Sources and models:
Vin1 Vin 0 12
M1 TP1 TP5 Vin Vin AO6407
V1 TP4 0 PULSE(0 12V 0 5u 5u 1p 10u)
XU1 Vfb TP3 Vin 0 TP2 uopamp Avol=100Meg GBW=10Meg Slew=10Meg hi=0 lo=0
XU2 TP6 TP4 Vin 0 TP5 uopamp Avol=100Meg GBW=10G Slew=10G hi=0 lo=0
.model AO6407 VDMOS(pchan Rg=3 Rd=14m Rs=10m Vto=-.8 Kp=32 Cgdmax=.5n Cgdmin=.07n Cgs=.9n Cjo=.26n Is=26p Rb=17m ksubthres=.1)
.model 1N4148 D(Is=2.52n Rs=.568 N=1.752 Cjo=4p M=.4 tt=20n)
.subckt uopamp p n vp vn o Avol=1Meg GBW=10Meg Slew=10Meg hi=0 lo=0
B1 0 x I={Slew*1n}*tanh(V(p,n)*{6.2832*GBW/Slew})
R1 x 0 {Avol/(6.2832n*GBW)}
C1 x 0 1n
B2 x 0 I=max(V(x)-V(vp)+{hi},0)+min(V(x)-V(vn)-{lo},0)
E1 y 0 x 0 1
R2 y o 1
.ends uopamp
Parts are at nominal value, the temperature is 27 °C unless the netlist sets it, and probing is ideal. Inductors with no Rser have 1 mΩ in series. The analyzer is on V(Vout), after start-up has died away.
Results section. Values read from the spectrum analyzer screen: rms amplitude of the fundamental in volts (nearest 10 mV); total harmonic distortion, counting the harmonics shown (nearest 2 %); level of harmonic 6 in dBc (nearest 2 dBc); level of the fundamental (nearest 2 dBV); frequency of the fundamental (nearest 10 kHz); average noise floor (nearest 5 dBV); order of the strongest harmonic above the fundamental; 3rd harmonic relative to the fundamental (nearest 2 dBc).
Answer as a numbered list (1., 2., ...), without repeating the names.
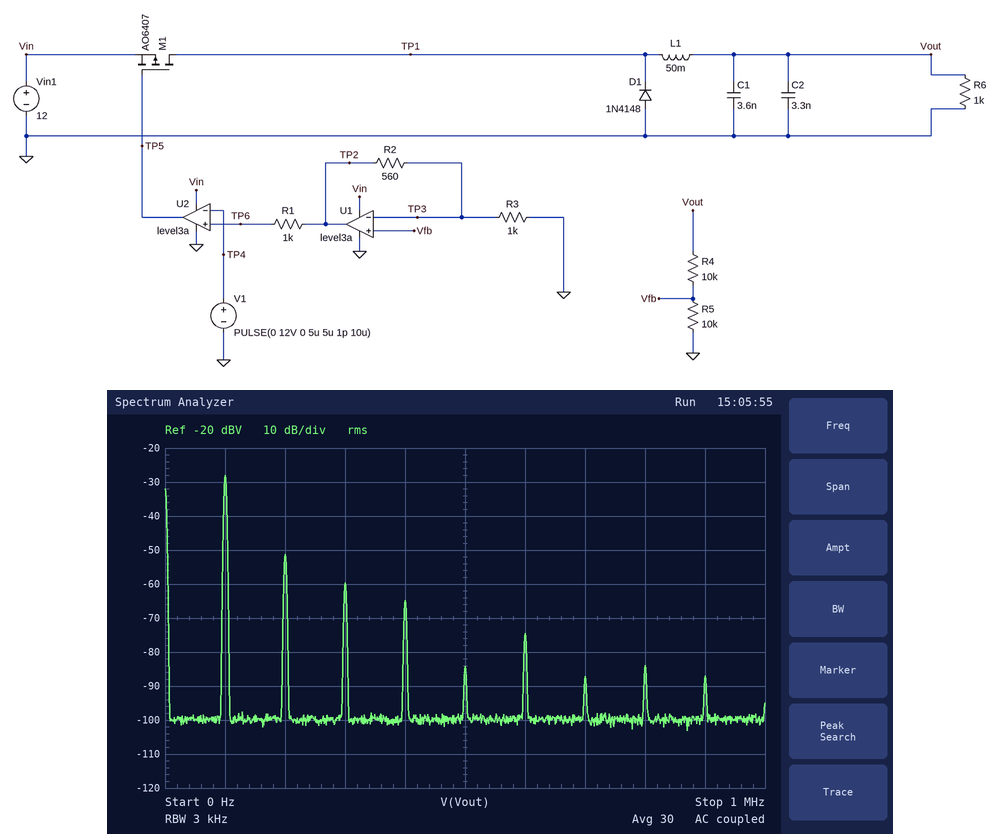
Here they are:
1. 40 mV
2. 8 %
3. -46 dBc
4. -28 dBV
5. 100 kHz
6. -100 dBV
7. 2
8. -32 dBc
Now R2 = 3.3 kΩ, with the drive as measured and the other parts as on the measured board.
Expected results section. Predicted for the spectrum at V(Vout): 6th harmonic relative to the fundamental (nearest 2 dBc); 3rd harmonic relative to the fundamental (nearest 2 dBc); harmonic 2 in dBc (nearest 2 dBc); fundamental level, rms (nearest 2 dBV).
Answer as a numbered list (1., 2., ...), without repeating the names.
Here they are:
1. -54 dBc
2. -40 dBc
3. -20 dBc
4. -28 dBV
